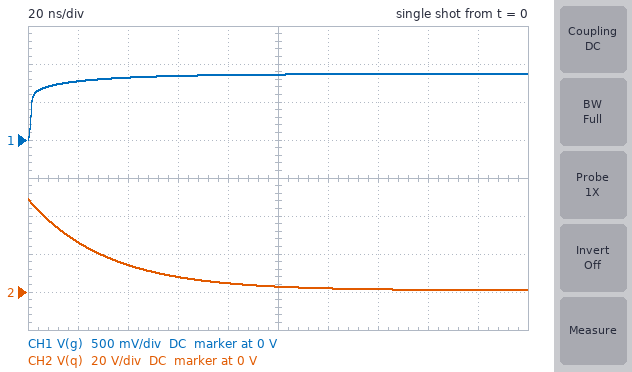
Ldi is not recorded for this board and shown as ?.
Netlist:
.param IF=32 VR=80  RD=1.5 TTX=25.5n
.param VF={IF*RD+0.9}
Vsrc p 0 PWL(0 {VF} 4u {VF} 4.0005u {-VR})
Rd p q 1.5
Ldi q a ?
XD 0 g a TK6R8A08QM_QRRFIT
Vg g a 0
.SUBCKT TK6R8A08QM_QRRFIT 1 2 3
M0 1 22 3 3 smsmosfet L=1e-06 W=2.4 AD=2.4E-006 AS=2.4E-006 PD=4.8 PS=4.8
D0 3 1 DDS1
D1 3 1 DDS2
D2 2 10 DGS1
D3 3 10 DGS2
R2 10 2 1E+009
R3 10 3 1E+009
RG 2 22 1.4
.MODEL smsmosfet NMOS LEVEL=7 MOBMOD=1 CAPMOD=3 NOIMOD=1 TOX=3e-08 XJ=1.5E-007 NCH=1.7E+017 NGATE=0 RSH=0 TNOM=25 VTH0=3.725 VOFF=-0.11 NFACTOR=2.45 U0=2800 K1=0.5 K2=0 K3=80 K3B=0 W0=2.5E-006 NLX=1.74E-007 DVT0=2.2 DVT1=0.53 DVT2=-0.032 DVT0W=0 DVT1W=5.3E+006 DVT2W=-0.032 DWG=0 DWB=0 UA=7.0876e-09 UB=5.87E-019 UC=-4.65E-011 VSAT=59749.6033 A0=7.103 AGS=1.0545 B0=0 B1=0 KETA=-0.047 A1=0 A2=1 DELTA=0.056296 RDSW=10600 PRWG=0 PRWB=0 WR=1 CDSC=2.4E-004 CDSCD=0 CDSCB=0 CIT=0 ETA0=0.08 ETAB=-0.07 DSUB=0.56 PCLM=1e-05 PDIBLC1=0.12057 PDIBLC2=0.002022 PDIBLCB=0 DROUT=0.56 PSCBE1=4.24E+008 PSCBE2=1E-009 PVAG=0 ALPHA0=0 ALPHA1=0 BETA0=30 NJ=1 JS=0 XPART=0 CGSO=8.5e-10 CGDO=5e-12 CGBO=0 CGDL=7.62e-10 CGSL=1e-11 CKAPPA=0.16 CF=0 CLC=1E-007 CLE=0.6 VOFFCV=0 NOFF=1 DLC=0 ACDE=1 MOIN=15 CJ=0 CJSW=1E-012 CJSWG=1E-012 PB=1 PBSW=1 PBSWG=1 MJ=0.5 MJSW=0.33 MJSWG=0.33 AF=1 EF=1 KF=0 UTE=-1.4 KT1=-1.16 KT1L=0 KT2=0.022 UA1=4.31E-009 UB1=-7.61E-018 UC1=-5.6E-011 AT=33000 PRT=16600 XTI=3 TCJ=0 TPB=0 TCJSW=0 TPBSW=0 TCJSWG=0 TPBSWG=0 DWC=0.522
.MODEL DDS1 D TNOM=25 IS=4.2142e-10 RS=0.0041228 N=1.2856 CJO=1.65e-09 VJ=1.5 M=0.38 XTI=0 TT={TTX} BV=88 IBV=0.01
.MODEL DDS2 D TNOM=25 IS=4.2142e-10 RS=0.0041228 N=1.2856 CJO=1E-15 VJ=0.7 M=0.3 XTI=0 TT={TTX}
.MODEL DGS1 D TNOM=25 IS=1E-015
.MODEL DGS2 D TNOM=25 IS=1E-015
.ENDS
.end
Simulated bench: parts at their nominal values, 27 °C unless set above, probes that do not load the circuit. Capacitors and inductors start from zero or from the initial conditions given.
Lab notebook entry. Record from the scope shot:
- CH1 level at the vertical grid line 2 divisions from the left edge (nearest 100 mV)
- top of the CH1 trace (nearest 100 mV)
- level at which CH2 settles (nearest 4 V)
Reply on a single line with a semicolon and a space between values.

800 mV; 900 mV; 0 V
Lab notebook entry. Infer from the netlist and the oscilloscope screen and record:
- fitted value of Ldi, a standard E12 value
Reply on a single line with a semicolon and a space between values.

47 nH
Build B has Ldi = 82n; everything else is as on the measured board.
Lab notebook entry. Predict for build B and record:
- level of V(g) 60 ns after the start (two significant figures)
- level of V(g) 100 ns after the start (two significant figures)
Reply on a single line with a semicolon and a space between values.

820 mV; 850 mV
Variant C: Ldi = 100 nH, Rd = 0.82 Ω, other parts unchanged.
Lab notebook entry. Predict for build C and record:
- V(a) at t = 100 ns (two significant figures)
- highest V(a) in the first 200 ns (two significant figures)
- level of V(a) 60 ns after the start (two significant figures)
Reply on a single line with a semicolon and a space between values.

860 mV; 910 mV; 820 mV
